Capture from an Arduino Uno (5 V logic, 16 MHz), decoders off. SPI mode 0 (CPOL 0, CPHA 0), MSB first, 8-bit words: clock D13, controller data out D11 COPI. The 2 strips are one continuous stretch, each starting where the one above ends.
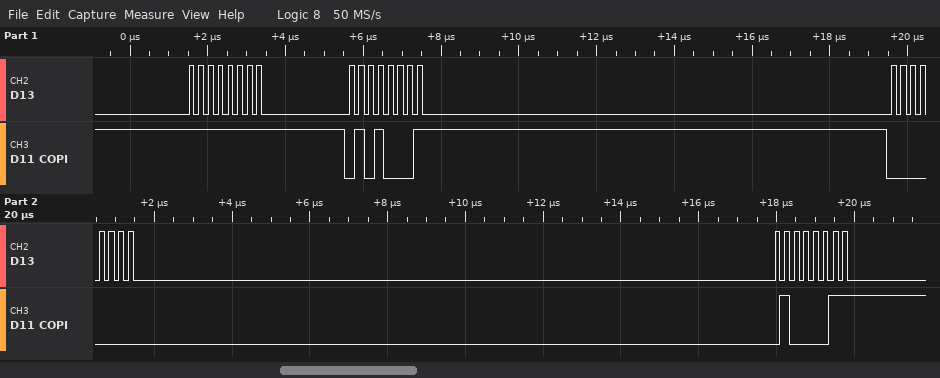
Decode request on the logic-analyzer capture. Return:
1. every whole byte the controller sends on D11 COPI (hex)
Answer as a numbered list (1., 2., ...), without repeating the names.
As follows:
1. 0xFF 0x51 0x00 0x43
